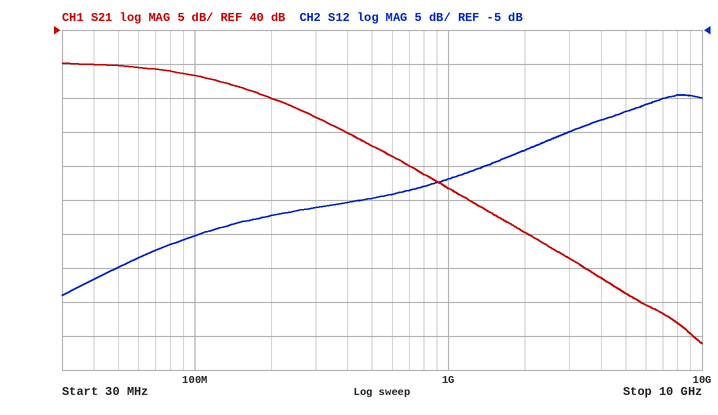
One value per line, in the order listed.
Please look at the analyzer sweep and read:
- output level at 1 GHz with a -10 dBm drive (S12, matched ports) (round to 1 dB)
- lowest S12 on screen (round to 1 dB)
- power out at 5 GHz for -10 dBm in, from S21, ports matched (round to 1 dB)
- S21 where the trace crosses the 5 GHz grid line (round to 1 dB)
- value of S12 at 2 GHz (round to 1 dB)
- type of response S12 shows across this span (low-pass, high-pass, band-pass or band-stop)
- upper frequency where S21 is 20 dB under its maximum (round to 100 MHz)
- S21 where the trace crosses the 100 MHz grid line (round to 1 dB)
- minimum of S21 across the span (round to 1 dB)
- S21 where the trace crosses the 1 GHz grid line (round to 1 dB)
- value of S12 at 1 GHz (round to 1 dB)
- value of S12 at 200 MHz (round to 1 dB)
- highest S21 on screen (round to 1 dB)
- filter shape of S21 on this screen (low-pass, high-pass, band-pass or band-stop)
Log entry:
-37 dBm
-44 dB
-9 dBm
1 dB
-23 dB
high-pass
1.2 GHz
33 dB
-6 dB
17 dB
-27 dB
-32 dB
35 dB
low-pass
